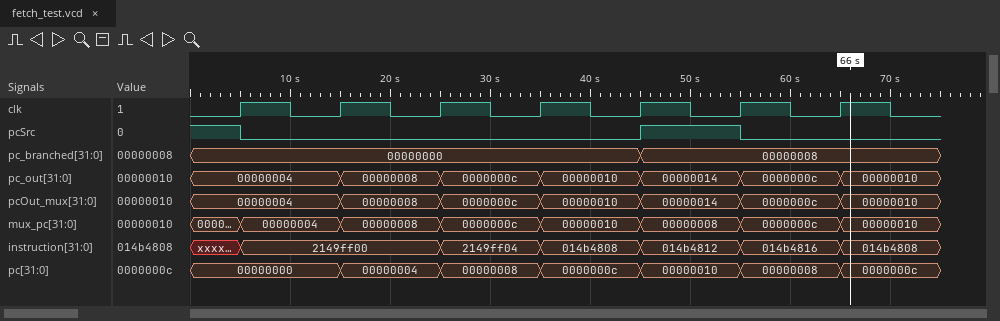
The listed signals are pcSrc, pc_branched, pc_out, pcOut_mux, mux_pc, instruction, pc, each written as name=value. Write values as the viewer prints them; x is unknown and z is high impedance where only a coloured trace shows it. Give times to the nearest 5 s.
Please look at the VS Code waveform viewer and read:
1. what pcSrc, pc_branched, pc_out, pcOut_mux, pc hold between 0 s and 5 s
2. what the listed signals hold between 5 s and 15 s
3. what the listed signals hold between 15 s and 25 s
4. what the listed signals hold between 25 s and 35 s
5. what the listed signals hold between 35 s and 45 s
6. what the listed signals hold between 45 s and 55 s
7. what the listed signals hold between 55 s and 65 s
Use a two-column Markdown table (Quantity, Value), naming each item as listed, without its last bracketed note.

| Quantity | Value |
|---|---|
| what pcSrc, pc_branched, pc_out, pcOut_mux, pc hold between 0 s and 5 s | pcSrc=1, pc_branched=00000000, pc_out=00000004, pcOut_mux=00000004, pc=00000000 |
| what the listed signals hold between 5 s and 15 s | pcSrc=0, pc_branched=00000000, pc_out=00000004, pcOut_mux=00000004, mux_pc=00000004, instruction=2149ff00, pc=00000000 |
| what the listed signals hold between 15 s and 25 s | pcSrc=0, pc_branched=00000000, pc_out=00000008, pcOut_mux=00000008, mux_pc=00000008, instruction=2149ff00, pc=00000004 |
| what the listed signals hold between 25 s and 35 s | pcSrc=0, pc_branched=00000000, pc_out=0000000c, pcOut_mux=0000000c, mux_pc=0000000c, instruction=2149ff04, pc=00000008 |
| what the listed signals hold between 35 s and 45 s | pcSrc=0, pc_branched=00000000, pc_out=00000010, pcOut_mux=00000010, mux_pc=00000010, instruction=014b4808, pc=0000000c |
| what the listed signals hold between 45 s and 55 s | pcSrc=1, pc_branched=00000008, pc_out=00000014, pcOut_mux=00000014, mux_pc=00000008, instruction=014b4812, pc=00000010 |
| what the listed signals hold between 55 s and 65 s | pcSrc=0, pc_branched=00000008, pc_out=0000000c, pcOut_mux=0000000c, mux_pc=0000000c, instruction=014b4816, pc=00000008 |
